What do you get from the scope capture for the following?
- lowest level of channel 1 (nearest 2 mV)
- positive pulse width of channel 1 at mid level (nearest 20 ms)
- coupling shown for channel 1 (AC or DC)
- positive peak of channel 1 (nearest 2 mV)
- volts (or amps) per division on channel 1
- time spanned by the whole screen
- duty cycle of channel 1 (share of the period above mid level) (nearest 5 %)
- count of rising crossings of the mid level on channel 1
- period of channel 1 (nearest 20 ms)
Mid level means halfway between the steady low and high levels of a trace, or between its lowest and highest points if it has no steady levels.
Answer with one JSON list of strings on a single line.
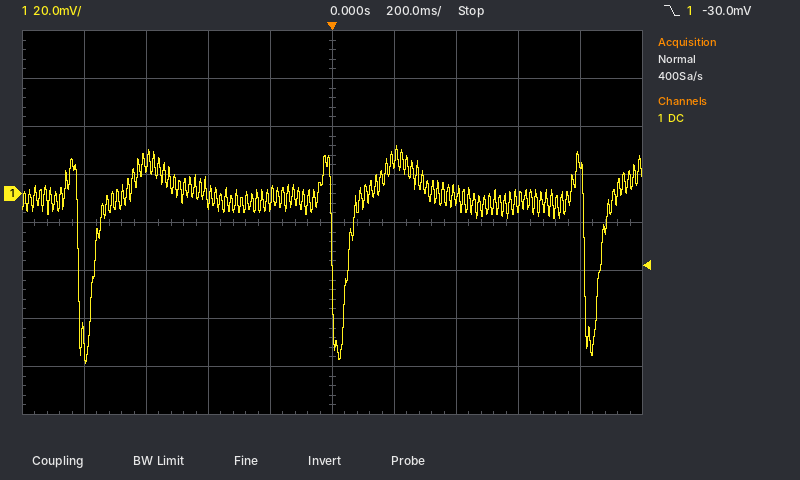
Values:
["-70 mV", "760 ms", "DC", "20 mV", "20 mV", "2 s", "95 %", "3", "820 ms"]
